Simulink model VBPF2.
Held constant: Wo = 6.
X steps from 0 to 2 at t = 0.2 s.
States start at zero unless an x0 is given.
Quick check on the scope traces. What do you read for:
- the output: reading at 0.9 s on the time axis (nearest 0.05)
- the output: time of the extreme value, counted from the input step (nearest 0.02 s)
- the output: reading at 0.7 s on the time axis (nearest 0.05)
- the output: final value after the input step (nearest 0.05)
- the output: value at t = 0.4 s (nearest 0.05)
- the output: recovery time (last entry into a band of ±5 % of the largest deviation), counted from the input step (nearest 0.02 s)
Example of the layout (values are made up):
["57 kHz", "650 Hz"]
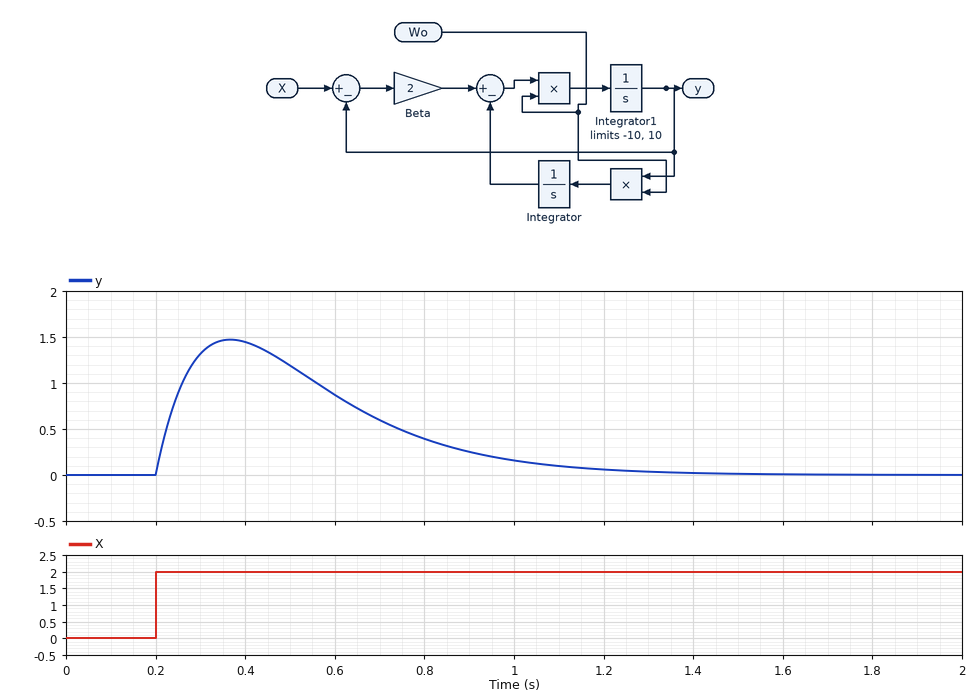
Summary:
["0.25", "0.16 s", "0.60", "0.00", "1.45", "0.96 s"]
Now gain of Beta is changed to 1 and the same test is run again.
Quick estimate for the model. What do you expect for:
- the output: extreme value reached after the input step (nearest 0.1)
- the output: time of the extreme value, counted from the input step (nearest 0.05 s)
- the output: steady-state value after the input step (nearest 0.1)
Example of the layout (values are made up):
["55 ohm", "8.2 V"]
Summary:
["1.1", "0.20 s", "0.0"]
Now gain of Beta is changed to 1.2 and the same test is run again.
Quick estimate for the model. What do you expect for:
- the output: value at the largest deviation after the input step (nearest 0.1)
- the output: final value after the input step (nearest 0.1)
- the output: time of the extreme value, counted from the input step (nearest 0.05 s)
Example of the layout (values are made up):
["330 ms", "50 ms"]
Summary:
["1.2", "0.0", "0.20 s"]
